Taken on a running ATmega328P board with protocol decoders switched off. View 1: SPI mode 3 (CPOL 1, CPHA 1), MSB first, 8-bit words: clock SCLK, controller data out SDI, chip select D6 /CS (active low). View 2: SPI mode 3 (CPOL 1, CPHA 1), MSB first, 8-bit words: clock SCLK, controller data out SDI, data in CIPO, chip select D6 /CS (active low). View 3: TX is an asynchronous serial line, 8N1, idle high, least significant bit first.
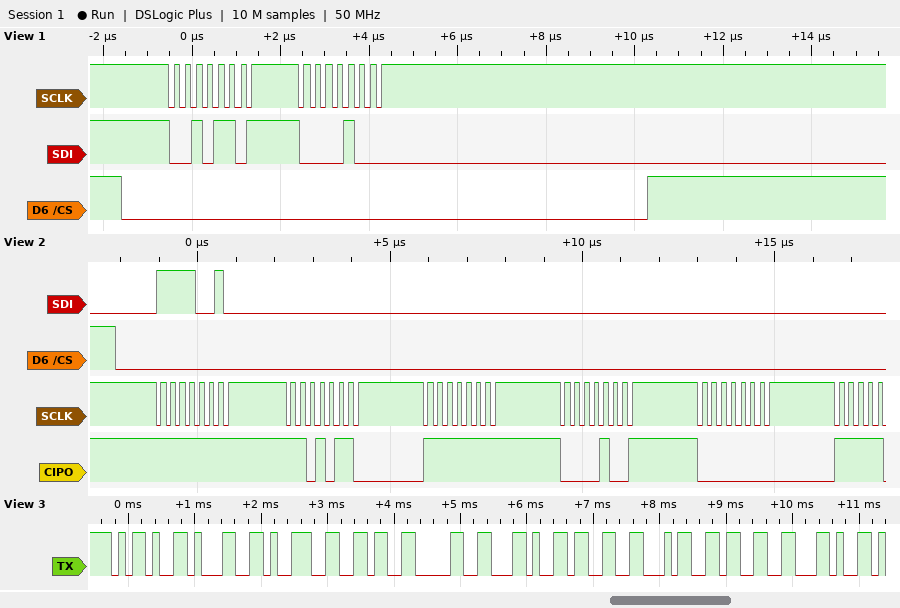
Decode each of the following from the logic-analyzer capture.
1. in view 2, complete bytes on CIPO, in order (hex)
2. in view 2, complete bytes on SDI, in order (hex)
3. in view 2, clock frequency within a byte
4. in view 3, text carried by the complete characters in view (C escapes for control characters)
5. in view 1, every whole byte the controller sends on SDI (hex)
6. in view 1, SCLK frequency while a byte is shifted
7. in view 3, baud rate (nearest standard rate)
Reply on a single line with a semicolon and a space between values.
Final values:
0xFF 0xD6 0xFF 0x09 0x00; 0xF2 0x00 0x00 0x00 0x00; 4 MHz; "-1960,343,"; 0x2D 0x08; 4 MHz; 9600 baud
